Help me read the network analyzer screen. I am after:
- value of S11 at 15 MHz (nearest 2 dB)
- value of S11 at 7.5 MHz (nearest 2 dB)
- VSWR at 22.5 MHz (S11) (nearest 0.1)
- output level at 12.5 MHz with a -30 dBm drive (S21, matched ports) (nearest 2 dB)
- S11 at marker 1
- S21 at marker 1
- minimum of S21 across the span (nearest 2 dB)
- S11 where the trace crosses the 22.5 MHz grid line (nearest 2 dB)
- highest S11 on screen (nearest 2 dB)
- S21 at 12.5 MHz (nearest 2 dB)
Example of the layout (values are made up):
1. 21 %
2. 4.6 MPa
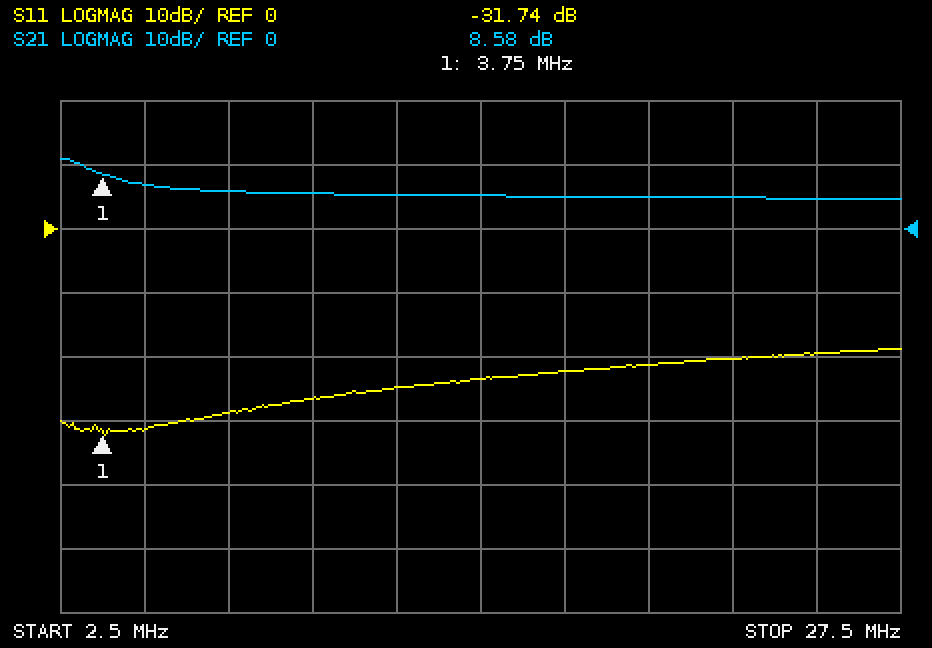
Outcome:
1. -24 dB
2. -28 dB
3. 1.2
4. -24 dBm
5. -31.74 dB
6. 8.58 dB
7. 4 dB
8. -20 dB
9. -18 dB
10. 6 dB
